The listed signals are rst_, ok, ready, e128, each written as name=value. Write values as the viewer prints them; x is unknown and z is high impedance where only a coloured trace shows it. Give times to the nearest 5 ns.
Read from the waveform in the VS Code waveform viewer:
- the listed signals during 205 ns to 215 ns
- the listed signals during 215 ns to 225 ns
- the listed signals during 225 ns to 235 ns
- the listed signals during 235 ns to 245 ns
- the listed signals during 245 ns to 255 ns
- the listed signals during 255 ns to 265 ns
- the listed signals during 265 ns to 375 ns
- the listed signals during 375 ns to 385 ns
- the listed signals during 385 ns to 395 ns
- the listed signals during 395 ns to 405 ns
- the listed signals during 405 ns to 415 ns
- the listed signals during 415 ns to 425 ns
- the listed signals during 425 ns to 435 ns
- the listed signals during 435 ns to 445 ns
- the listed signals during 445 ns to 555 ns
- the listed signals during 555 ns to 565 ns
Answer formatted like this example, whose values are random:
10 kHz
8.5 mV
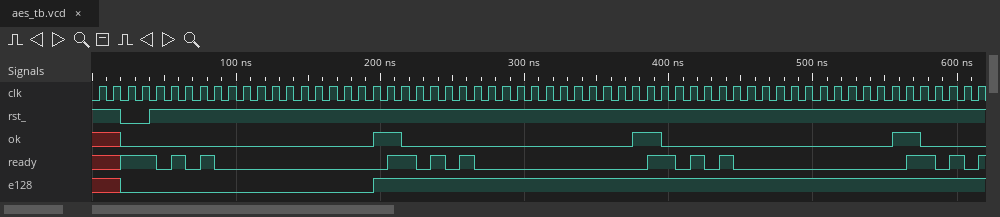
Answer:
rst_=1, ok=1, ready=1, e128=1
rst_=1, ok=0, ready=1, e128=1
rst_=1, ok=0, ready=0, e128=1
rst_=1, ok=0, ready=1, e128=1
rst_=1, ok=0, ready=0, e128=1
rst_=1, ok=0, ready=1, e128=1
rst_=1, ok=0, ready=0, e128=1
rst_=1, ok=1, ready=0, e128=1
rst_=1, ok=1, ready=1, e128=1
rst_=1, ok=0, ready=1, e128=1
rst_=1, ok=0, ready=0, e128=1
rst_=1, ok=0, ready=1, e128=1
rst_=1, ok=0, ready=0, e128=1
rst_=1, ok=0, ready=1, e128=1
rst_=1, ok=0, ready=0, e128=1
rst_=1, ok=1, ready=0, e128=1
